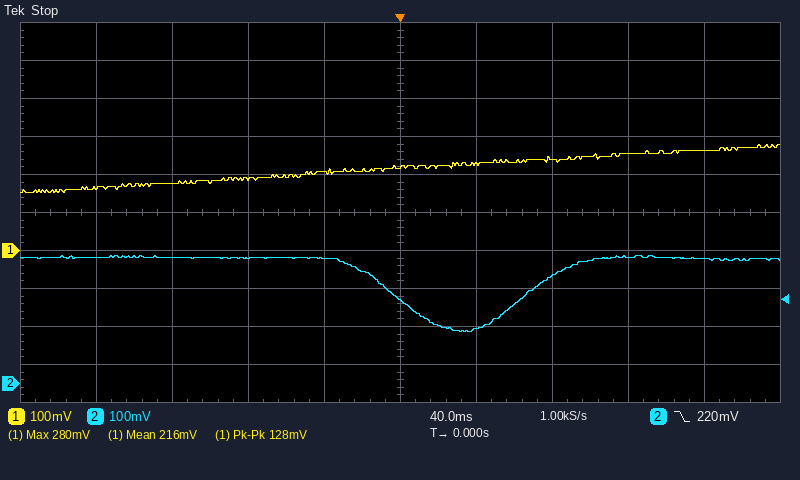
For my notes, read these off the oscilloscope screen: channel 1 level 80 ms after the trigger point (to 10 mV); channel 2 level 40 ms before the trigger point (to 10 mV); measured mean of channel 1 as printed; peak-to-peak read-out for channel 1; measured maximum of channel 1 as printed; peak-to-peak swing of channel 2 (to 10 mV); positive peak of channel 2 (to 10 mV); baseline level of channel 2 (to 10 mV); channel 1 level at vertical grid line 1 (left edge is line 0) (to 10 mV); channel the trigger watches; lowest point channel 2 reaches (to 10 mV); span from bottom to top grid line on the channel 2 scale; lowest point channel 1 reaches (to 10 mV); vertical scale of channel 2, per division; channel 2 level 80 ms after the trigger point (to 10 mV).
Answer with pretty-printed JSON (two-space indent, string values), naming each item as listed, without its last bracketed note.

{
  "channel 1 level 80 ms after the trigger point": "240 mV",
  "channel 2 level 40 ms before the trigger point": "330 mV",
  "measured mean of channel 1 as printed": "216 mV",
  "peak-to-peak read-out for channel 1": "128 mV",
  "measured maximum of channel 1 as printed": "280 mV",
  "peak-to-peak swing of channel 2": "200 mV",
  "positive peak of channel 2": "340 mV",
  "baseline level of channel 2": "330 mV",
  "channel 1 level at vertical grid line 1 (left edge is line 0)": "160 mV",
  "channel the trigger watches": "channel 2",
  "lowest point channel 2 reaches": "140 mV",
  "span from bottom to top grid line on the channel 2 scale": "1 V",
  "lowest point channel 1 reaches": "150 mV",
  "vertical scale of channel 2, per division": "100 mV",
  "channel 2 level 80 ms after the trigger point": "280 mV"
}
